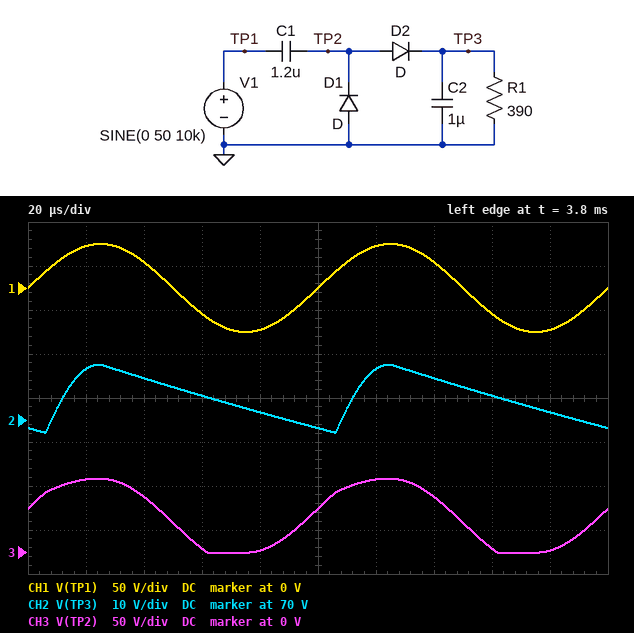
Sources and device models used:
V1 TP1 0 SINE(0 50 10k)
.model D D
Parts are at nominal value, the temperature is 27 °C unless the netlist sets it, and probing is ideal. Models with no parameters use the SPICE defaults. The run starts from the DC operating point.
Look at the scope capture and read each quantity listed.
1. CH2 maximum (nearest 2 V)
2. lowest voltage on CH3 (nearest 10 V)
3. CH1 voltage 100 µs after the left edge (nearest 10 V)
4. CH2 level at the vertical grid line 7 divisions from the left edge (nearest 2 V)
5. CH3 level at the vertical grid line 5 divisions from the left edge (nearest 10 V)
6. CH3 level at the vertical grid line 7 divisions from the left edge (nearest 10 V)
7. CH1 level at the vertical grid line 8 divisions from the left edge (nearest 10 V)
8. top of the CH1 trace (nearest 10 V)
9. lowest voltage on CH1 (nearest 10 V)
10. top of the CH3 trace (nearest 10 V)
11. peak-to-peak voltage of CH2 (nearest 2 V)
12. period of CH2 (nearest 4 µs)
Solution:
82 V
0 V
0 V
80 V
50 V
60 V
-30 V
50 V
-50 V
80 V
16 V
100 µs
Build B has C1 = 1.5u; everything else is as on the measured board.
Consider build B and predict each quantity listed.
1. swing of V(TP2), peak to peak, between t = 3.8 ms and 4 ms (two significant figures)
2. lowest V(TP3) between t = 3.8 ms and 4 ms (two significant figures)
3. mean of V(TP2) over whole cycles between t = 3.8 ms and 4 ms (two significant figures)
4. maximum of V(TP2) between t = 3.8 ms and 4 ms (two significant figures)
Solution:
87 V
69 V
42 V
86 V
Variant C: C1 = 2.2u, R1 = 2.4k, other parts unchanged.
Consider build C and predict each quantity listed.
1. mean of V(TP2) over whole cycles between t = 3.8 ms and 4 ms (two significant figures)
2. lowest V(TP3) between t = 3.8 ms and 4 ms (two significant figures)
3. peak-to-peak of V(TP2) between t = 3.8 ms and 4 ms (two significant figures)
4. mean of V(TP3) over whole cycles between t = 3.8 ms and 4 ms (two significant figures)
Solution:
48 V
93 V
98 V
95 V
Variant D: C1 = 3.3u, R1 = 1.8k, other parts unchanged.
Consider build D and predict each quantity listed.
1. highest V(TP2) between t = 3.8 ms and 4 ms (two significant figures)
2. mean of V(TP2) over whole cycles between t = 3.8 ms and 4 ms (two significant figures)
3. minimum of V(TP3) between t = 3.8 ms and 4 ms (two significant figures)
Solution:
98 V
48 V
92 V
